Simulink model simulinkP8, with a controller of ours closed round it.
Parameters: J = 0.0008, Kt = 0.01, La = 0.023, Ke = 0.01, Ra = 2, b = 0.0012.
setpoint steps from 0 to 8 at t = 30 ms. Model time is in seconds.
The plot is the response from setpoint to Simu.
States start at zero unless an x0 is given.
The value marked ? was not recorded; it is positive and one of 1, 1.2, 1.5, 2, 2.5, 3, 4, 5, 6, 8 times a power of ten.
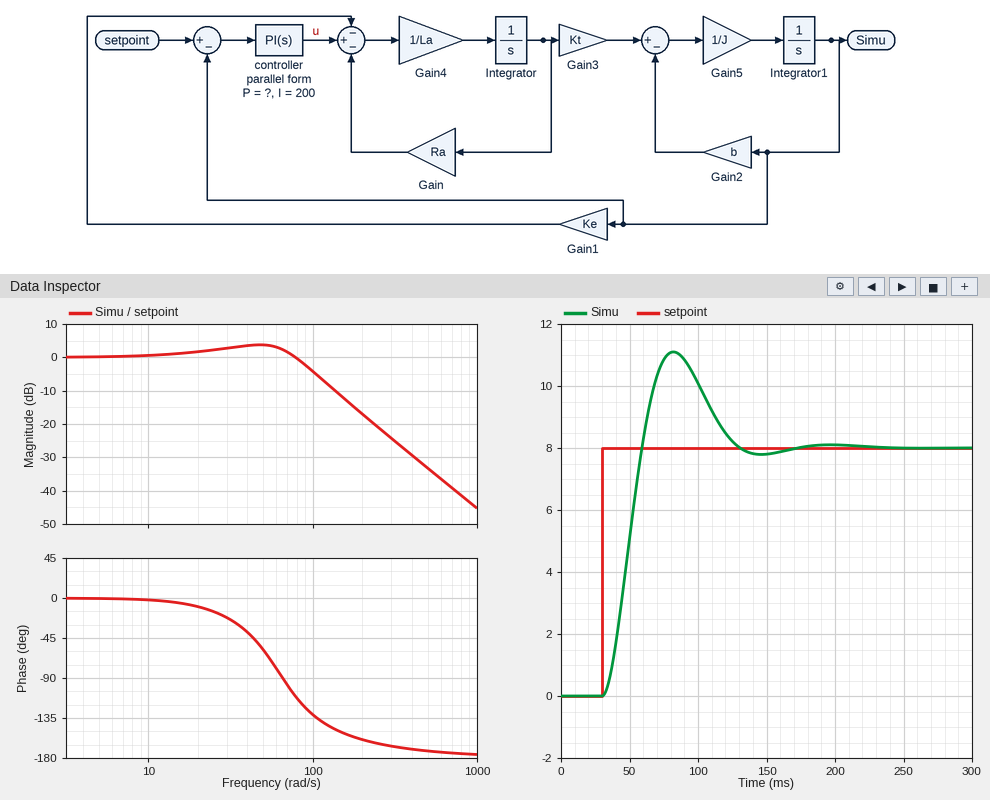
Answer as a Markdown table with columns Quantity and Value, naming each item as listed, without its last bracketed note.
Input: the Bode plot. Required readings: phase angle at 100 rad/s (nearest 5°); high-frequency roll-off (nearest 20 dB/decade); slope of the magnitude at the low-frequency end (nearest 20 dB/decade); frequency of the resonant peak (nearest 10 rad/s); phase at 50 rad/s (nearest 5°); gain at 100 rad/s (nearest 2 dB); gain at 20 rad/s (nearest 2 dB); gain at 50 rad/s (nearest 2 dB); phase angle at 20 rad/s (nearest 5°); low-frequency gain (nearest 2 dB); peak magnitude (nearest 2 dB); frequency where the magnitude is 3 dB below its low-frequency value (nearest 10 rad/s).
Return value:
| Quantity | Value |
|---|---|
| phase angle at 100 rad/s | -130° |
| high-frequency roll-off | -40 dB/decade |
| slope of the magnitude at the low-frequency end | 0 dB/decade |
| frequency of the resonant peak | 50 rad/s |
| phase at 50 rad/s | -60° |
| gain at 100 rad/s | -4 dB |
| gain at 20 rad/s | 2 dB |
| gain at 50 rad/s | 4 dB |
| phase angle at 20 rad/s | -10° |
| low-frequency gain | 0 dB |
| peak magnitude | 4 dB |
| frequency where the magnitude is 3 dB below its low-frequency value | 90 rad/s |
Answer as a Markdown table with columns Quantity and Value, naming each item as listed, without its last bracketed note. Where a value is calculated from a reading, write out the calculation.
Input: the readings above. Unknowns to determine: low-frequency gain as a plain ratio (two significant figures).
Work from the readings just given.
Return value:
| Quantity | Value |
|---|---|
| low-frequency gain as a plain ratio | 10^(0 / 20) = 1.0 |
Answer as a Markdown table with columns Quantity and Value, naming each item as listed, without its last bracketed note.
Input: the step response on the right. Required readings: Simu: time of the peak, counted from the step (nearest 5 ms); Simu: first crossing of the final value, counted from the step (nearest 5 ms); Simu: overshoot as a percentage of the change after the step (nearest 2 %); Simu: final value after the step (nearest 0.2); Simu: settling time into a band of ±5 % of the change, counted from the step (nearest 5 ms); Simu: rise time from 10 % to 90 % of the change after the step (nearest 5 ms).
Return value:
| Quantity | Value |
|---|---|
| Simu: time of the peak, counted from the step | 50 ms |
| Simu: first crossing of the final value, counted from the step | 30 ms |
| Simu: overshoot as a percentage of the change after the step | 38 % |
| Simu: final value after the step | 8.0 |
| Simu: settling time into a band of ±5 % of the change, counted from the step | 90 ms |
| Simu: rise time from 10 % to 90 % of the change after the step | 20 ms |
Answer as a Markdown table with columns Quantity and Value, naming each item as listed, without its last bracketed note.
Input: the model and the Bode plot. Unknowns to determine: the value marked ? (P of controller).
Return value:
| Quantity | Value |
|---|---|
| the value marked ? | 10 |
